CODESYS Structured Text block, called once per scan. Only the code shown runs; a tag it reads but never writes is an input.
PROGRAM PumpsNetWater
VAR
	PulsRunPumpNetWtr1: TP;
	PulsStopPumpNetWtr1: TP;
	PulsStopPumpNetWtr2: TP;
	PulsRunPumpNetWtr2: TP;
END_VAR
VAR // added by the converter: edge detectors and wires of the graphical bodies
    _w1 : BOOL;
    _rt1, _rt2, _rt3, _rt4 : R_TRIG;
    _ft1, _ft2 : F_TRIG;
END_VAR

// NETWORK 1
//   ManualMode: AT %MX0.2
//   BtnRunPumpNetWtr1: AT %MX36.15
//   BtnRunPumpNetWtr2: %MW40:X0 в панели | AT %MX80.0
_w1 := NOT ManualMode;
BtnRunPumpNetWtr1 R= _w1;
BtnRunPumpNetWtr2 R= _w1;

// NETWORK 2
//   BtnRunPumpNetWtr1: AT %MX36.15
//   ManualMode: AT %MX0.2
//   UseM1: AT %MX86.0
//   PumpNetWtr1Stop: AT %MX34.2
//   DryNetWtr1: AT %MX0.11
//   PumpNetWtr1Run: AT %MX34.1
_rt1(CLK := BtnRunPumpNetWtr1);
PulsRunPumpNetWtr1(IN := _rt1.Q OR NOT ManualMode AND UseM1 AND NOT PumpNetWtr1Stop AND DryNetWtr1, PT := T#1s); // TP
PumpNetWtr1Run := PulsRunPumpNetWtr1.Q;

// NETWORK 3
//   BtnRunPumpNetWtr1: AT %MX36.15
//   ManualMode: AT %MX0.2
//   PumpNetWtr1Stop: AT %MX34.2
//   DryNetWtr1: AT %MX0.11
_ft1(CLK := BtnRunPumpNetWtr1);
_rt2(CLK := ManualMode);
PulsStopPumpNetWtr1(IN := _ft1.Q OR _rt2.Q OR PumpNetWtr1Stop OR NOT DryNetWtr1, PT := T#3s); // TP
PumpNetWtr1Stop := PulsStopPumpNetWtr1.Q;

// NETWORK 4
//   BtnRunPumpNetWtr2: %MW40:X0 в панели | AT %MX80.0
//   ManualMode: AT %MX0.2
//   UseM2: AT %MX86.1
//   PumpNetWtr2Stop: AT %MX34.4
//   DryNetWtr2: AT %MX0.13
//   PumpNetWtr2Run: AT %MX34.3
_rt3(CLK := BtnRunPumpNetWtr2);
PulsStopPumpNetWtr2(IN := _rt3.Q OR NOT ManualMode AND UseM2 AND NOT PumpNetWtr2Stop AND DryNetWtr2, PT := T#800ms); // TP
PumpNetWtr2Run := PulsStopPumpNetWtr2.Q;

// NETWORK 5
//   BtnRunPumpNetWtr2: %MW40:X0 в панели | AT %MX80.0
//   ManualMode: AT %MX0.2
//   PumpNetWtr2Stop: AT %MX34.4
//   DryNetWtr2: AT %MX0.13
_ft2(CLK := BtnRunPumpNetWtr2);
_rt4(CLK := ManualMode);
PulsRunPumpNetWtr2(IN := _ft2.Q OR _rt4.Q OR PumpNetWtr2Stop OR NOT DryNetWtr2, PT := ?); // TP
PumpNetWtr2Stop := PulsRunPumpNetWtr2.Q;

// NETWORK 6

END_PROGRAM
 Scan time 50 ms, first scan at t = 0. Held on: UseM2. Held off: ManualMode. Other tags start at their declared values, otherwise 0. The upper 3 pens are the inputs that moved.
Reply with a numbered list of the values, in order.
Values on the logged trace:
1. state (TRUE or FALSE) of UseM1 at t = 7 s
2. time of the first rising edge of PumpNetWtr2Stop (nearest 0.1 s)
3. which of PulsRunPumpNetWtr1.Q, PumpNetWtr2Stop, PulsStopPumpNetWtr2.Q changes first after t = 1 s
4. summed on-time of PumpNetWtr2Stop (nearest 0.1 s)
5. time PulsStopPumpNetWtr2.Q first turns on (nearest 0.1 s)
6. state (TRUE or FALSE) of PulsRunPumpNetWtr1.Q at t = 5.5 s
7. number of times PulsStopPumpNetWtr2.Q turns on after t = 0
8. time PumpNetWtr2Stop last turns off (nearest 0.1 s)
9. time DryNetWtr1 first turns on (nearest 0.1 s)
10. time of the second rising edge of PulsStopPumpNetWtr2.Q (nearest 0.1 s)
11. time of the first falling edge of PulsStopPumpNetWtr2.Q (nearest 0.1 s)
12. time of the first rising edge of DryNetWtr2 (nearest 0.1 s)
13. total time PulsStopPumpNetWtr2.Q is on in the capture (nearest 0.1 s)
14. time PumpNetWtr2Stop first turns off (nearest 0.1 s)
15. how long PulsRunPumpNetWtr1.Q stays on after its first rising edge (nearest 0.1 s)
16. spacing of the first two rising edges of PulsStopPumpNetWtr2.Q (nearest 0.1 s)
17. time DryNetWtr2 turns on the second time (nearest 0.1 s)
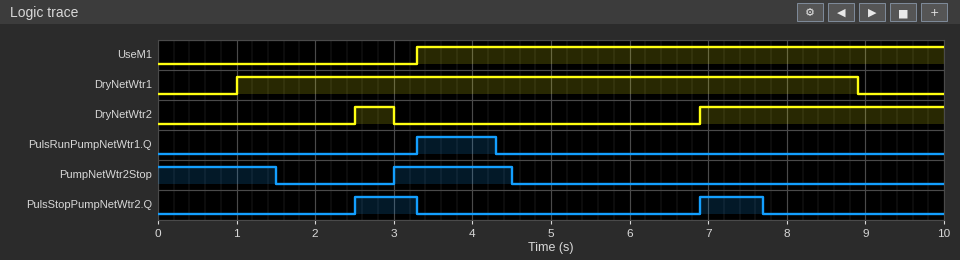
1. TRUE
2. 3.0 s
3. PumpNetWtr2Stop
4. 3.0 s
5. 2.5 s
6. FALSE
7. 2
8. 4.5 s
9. 1.0 s
10. 6.9 s
11. 3.3 s
12. 2.5 s
13. 1.6 s
14. 1.5 s
15. 1.0 s
16. 4.4 s
17. 6.9 s
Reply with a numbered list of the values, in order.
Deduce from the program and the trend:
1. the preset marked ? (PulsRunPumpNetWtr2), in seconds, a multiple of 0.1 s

1. 1.5 s
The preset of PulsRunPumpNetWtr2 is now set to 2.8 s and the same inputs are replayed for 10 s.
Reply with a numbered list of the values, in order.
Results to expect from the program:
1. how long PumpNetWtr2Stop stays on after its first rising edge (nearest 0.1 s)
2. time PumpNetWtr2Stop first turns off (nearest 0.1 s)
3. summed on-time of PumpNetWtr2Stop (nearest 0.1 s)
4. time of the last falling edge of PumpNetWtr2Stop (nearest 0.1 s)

1. 2.8 s
2. 2.8 s
3. 5.6 s
4. 5.8 s
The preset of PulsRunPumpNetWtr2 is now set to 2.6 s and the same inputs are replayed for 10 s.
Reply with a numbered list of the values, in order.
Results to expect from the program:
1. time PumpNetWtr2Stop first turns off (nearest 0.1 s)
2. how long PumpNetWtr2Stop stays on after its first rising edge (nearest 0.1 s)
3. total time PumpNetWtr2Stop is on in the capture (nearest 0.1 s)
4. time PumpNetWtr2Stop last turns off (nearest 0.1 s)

1. 2.6 s
2. 2.6 s
3. 5.2 s
4. 5.6 s
